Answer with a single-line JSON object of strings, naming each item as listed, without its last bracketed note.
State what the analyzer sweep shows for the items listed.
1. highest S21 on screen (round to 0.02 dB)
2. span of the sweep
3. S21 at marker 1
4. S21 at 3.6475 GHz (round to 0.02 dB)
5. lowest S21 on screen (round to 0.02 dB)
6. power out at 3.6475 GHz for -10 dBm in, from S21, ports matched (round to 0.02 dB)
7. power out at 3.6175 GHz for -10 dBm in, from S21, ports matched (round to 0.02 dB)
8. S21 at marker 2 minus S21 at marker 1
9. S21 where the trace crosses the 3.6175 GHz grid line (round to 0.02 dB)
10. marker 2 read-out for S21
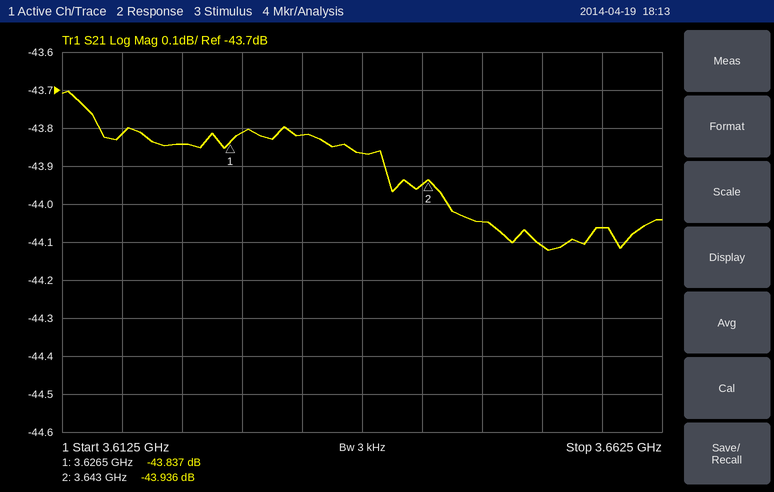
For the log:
{"highest S21 on screen": "-43.70 dB", "span of the sweep": "50 MHz", "S21 at marker 1": "-43.837 dB", "S21 at 3.6475 GHz": "-44.04 dB", "lowest S21 on screen": "-44.12 dB", "power out at 3.6475 GHz for -10 dBm in, from S21, ports matched": "-54.04 dBm", "power out at 3.6175 GHz for -10 dBm in, from S21, ports matched": "-53.82 dBm", "S21 at marker 2 minus S21 at marker 1": "-0.099 dB", "S21 where the trace crosses the 3.6175 GHz grid line": "-43.82 dB", "marker 2 read-out for S21": "-43.936 dB"}
